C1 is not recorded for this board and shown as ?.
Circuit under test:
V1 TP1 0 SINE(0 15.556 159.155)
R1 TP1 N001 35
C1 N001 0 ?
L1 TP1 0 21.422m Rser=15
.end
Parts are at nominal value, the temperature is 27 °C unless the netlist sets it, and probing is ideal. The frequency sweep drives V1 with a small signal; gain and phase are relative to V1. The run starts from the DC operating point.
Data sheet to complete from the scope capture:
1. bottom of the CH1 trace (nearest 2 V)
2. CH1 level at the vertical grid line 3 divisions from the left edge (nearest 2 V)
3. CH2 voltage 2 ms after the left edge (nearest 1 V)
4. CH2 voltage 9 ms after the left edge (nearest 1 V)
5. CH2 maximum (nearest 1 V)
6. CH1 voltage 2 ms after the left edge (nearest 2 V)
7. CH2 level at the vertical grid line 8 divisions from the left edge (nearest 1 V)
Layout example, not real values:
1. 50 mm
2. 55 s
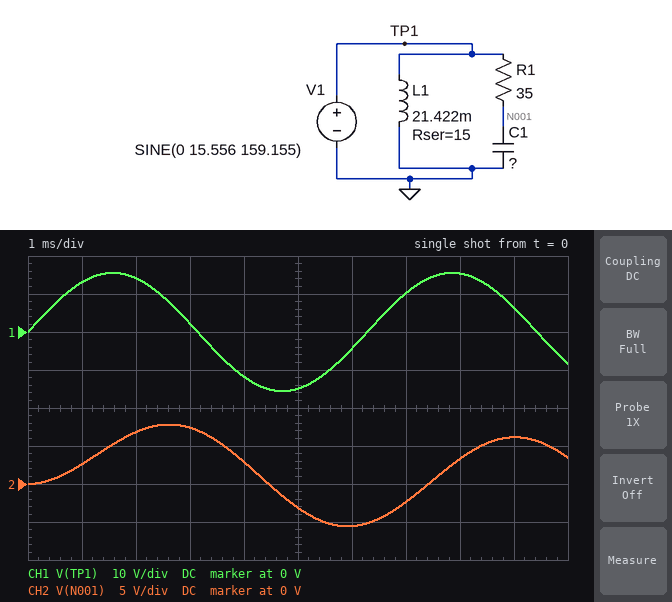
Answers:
1. -16 V
2. 2 V
3. 7 V
4. 6 V
5. 8 V
6. 14 V
7. 3 V
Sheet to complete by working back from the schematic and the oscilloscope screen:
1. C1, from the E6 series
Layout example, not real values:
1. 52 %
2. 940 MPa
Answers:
1. 68 µF
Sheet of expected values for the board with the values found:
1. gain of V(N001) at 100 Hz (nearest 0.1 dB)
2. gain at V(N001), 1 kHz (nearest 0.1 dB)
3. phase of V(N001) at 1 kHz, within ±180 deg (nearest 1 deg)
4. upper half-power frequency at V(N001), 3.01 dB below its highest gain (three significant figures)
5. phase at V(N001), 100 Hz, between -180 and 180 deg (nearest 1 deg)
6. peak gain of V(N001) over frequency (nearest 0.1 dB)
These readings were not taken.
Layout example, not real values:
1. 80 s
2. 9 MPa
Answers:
1. -5.1 dB
2. -23.5 dB
3. -86 deg
4. 66.9 Hz
5. -56 deg
6. 0 dB
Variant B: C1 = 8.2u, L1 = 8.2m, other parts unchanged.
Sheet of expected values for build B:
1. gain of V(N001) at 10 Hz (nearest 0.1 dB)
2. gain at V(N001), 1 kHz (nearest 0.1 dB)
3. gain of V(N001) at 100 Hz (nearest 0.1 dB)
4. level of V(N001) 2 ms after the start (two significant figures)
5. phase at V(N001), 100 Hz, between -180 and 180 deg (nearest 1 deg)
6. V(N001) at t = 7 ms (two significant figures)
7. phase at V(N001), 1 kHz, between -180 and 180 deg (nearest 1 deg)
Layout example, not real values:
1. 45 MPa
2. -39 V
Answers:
1. 0 dB
2. -6.3 dB
3. -0.1 dB
4. 15 V
5. -10 deg
6. 6.3 V
7. -61 deg
